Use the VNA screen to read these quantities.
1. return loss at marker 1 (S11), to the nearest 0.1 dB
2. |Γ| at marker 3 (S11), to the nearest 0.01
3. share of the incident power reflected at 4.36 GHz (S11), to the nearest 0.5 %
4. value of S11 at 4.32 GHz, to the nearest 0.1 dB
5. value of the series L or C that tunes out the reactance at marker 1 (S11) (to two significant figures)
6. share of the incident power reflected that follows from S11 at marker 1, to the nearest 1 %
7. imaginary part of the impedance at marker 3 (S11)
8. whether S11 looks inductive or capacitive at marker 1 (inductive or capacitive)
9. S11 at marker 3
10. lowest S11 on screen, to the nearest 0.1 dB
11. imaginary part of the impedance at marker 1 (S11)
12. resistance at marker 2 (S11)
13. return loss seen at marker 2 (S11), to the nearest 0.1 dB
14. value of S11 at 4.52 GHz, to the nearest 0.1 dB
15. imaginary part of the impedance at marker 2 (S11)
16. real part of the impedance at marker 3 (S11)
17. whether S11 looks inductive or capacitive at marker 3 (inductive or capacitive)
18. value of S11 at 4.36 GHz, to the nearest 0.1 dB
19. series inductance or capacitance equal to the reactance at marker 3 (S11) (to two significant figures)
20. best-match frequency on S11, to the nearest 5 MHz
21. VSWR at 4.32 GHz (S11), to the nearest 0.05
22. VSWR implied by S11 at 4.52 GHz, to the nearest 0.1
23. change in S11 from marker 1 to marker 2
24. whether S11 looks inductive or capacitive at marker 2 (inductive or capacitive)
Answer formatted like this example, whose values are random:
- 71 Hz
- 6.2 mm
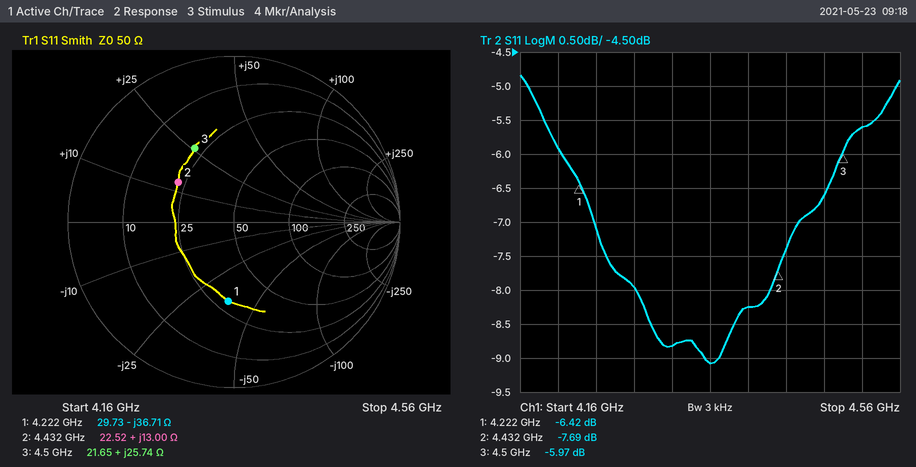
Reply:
- 6.4 dB
- 0.50
- 12.5 %
- -8.8 dB
- 1.4 nH
- 23 %
- +25.74 Ω
- capacitive
- -5.97 dB
- -9.1 dB
- -36.71 Ω
- 22.52 Ω
- 7.7 dB
- -5.6 dB
- +13.00 Ω
- 21.65 Ω
- inductive
- -9.1 dB
- 910 pH
- 4.360 GHz
- 2.15
- 3.2
- -1.27 dB
- inductive
